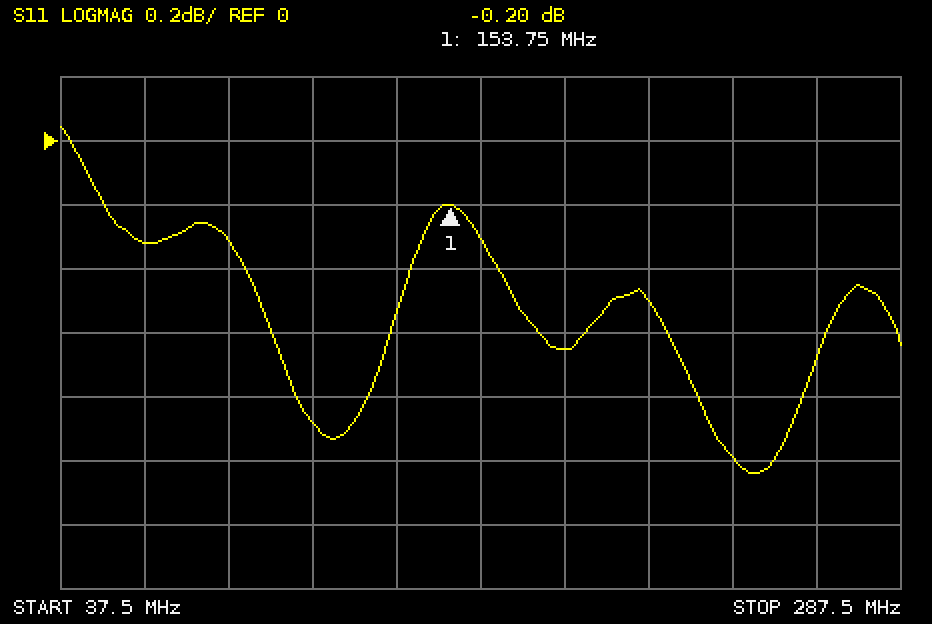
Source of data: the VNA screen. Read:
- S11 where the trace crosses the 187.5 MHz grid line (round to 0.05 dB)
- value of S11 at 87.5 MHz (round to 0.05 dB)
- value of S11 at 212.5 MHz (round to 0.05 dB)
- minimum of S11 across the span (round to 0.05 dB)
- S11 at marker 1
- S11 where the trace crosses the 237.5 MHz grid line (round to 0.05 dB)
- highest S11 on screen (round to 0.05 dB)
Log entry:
-0.65 dB
-0.30 dB
-0.50 dB
-1.05 dB
-0.20 dB
-1.00 dB
0.05 dB
